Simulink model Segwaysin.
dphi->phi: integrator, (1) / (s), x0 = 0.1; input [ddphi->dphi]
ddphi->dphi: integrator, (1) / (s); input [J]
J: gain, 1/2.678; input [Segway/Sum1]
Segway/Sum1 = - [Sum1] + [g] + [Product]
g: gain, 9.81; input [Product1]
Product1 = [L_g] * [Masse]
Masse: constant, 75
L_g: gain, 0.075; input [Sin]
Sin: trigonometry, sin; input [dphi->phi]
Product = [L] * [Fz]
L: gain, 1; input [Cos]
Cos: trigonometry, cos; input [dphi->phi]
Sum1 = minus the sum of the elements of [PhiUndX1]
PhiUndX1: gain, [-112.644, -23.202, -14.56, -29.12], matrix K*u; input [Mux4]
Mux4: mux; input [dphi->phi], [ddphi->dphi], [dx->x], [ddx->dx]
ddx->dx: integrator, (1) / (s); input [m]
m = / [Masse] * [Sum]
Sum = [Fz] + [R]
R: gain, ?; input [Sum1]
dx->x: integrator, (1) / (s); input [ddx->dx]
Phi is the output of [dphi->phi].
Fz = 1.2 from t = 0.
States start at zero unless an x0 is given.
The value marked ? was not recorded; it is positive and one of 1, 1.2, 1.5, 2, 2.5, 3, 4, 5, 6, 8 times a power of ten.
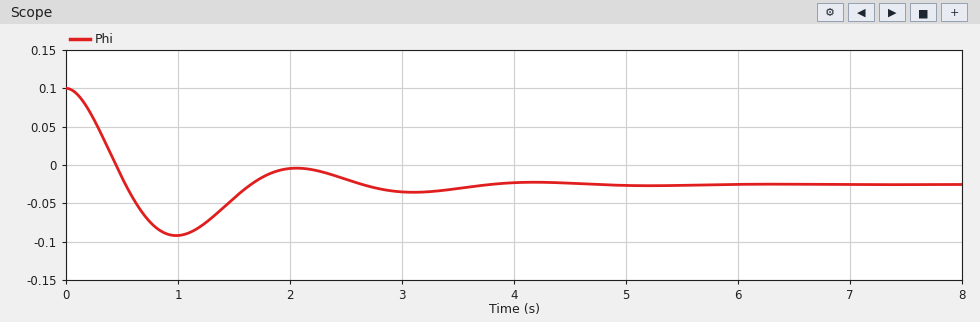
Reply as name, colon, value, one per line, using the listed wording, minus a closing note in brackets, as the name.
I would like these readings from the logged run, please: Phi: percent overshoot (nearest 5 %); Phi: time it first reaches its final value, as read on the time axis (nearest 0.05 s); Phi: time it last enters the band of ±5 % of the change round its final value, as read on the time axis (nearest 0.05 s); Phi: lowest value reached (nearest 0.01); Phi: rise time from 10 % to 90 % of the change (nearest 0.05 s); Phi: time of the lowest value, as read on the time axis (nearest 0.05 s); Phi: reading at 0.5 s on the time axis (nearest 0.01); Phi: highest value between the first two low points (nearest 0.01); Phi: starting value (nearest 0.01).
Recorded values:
Phi: percent overshoot: 55 %
Phi: time it first reaches its final value, as read on the time axis: 0.55 s
Phi: time it last enters the band of ±5 % of the change round its final value, as read on the time axis: 3.45 s
Phi: lowest value reached: -0.09
Phi: rise time from 10 % to 90 % of the change: 0.35 s
Phi: time of the lowest value, as read on the time axis: 1.00 s
Phi: reading at 0.5 s on the time axis: -0.02
Phi: highest value between the first two low points: 0.00
Phi: starting value: 0.10
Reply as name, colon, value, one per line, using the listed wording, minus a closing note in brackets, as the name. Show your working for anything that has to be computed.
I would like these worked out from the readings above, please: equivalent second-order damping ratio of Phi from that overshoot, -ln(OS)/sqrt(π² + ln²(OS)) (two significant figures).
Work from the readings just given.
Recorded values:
equivalent second-order damping ratio of Phi from that overshoot, -ln(OS)/sqrt(π² + ln²(OS)): ln(0.55) = -0.598; 0.598 / sqrt(9.870 + 0.357) = 0.19
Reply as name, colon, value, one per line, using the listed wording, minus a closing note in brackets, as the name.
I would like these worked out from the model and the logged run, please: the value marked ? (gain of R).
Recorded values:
the value marked ?: 6
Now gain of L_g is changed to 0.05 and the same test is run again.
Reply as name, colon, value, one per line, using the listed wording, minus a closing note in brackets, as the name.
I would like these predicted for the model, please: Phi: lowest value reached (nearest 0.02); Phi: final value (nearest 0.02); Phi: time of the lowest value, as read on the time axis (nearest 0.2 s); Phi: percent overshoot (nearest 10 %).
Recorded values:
Phi: lowest value reached: -0.06
Phi: final value: -0.04
Phi: time of the lowest value, as read on the time axis: 1.0 s
Phi: percent overshoot: 20 %
